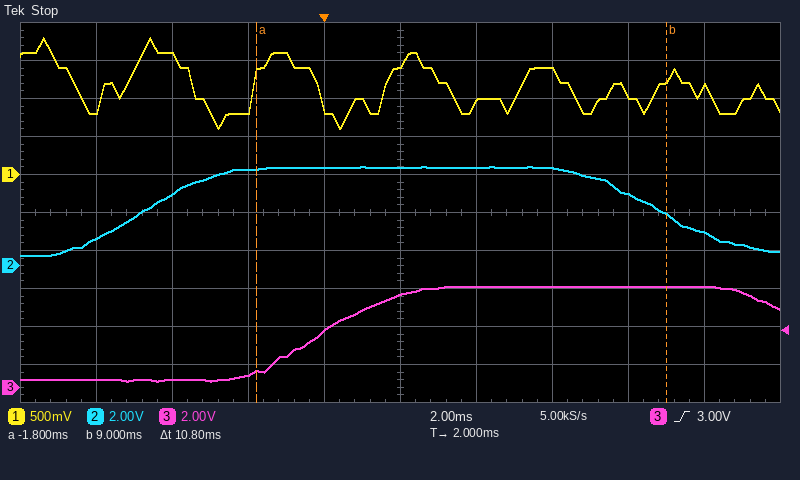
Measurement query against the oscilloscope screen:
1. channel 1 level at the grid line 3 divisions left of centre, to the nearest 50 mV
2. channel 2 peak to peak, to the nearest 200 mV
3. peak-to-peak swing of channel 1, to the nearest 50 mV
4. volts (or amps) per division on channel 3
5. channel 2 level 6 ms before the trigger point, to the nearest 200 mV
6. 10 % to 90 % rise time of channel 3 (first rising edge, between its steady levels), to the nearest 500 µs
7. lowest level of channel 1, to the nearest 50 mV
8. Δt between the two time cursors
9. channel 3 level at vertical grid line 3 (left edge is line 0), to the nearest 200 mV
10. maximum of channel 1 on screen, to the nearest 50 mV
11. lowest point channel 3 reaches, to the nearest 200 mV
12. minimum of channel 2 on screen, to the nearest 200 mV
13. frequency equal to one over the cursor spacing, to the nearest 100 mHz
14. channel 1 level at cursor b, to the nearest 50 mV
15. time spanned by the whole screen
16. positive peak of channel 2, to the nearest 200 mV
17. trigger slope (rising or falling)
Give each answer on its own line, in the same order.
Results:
1.55 V
4.6 V
1.20 V
2 V
1.4 V
3.5 ms
600 mV
10.8 ms
600 mV
1.80 V
400 mV
600 mV
92.6 Hz
1.25 V
20 ms
5.2 V
rising
